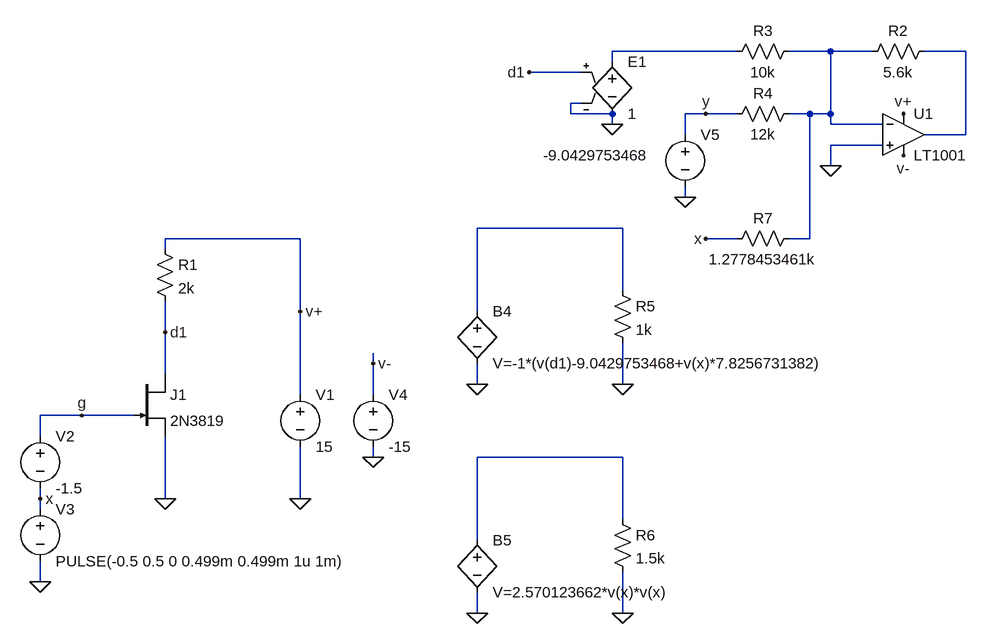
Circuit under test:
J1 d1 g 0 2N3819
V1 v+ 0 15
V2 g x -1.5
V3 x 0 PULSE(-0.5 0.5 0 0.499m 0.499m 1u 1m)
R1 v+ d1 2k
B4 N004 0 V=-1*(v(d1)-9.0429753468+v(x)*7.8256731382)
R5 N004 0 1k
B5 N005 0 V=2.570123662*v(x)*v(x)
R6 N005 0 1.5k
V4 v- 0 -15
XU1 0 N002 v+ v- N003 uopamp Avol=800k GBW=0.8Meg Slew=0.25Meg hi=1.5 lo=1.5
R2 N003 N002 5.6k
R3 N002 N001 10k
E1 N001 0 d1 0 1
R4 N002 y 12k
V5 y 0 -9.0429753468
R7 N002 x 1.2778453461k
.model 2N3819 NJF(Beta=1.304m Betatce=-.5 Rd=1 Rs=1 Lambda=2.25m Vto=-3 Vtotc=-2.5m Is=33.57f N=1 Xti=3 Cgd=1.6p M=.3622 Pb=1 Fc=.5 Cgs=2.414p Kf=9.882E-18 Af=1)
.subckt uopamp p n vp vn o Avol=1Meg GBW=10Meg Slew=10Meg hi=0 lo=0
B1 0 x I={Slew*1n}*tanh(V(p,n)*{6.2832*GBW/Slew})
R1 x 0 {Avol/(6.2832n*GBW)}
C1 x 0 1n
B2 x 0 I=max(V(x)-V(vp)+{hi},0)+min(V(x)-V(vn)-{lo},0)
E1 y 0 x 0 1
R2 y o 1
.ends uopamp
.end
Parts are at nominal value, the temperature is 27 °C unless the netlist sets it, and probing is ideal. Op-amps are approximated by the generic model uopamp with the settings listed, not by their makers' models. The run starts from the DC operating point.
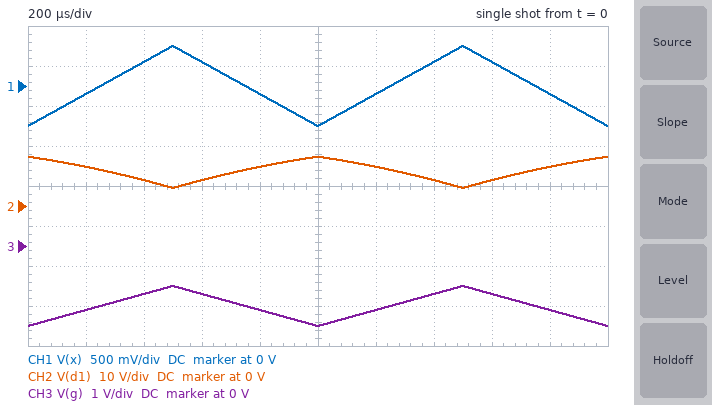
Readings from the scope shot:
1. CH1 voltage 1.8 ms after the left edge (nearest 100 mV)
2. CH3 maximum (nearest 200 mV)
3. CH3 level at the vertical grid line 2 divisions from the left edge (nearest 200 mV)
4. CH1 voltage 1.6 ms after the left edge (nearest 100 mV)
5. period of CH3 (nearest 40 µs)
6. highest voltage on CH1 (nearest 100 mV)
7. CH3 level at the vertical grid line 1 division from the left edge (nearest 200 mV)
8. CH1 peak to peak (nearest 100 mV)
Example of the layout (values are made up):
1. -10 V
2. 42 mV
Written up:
1. -100 mV
2. -1.0 V
3. -1.2 V
4. 300 mV
5. 1.00 ms
6. 500 mV
7. -1.6 V
8. 1.0 V
